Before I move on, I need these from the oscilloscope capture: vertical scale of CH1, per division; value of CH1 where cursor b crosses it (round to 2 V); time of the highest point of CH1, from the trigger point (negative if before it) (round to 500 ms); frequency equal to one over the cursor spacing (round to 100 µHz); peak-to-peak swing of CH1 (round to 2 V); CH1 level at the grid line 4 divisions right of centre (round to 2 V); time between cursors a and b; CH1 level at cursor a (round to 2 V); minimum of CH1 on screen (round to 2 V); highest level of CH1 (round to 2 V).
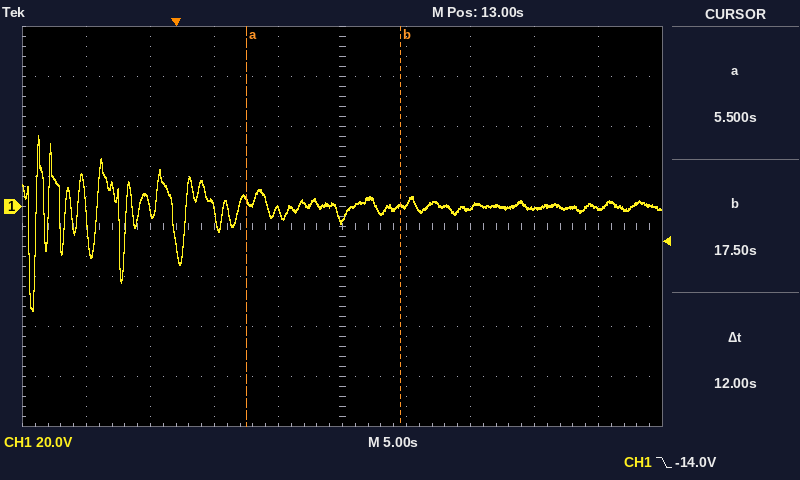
20 V
0 V
-10.5 s
83.3 mHz
70 V
0 V
12 s
2 V
-42 V
28 V
